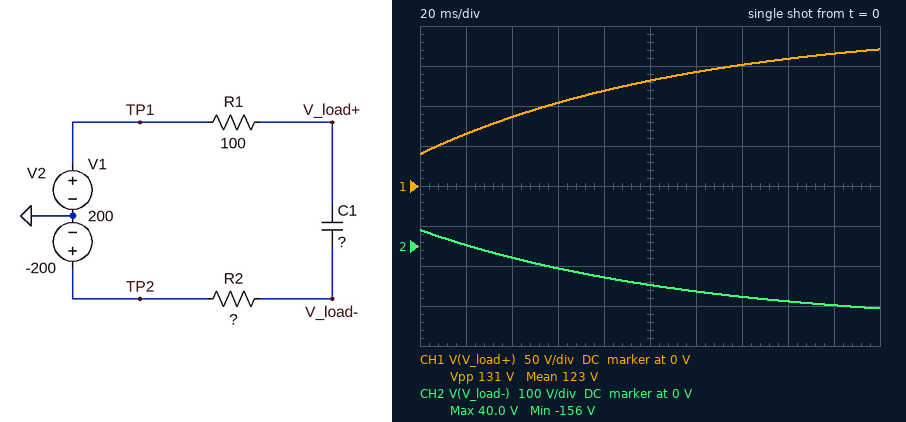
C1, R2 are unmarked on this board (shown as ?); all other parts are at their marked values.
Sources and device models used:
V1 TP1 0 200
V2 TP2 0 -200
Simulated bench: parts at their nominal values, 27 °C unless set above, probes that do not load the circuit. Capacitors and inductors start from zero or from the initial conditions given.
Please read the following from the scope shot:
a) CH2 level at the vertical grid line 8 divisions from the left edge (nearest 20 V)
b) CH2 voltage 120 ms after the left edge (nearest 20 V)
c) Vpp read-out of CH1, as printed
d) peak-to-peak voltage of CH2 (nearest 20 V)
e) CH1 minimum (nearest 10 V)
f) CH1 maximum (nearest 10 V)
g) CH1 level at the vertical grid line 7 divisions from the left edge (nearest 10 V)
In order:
-140 V
-120 V
131 V
200 V
40 V
170 V
150 V
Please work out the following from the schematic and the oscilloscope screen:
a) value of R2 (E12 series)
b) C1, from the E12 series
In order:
150 Ω
470 µF
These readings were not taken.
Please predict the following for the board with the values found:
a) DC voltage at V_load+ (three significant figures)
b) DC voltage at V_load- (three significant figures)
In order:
200 V
-200 V
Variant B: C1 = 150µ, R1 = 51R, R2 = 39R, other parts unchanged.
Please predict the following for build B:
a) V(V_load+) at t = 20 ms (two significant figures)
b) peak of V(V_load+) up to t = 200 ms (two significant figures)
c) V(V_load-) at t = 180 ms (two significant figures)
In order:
150 V
200 V
-200 V
